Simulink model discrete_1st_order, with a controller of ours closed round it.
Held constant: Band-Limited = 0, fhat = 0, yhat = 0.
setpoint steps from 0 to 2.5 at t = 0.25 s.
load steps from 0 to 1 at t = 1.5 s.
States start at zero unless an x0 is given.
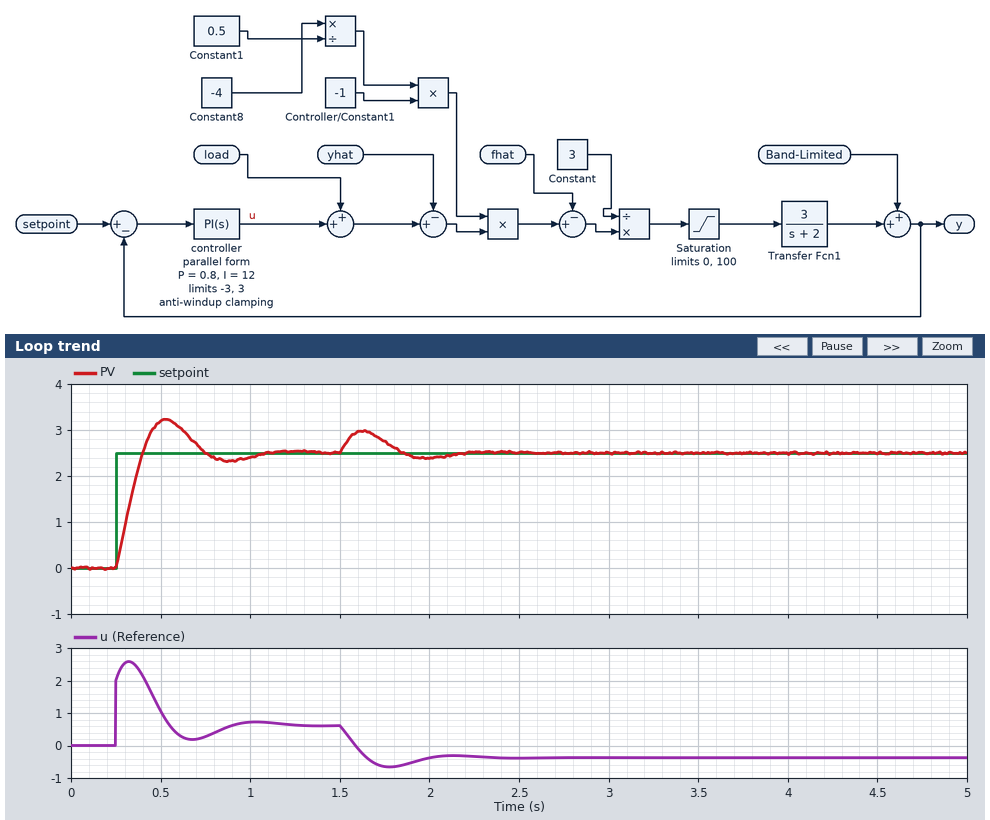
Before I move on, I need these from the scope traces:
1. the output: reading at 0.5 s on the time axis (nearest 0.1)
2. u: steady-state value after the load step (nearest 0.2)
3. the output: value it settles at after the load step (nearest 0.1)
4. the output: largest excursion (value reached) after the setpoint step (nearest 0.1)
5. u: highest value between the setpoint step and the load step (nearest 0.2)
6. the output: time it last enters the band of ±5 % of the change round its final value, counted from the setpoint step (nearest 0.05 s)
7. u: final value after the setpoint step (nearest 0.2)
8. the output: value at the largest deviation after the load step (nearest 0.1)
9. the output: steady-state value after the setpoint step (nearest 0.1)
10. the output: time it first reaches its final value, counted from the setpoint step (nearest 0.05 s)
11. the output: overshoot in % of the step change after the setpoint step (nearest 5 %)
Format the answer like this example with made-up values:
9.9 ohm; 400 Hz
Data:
3.2; -0.4; 2.5; 3.2; 2.6; 0.70 s; 0.6; 3.0; 2.5; 0.15 s; 30 %
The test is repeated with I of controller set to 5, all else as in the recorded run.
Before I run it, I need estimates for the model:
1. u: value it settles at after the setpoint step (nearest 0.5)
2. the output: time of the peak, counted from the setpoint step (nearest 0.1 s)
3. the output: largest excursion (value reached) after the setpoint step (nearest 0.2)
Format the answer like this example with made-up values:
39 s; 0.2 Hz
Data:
0.5; 0.4 s; 2.8
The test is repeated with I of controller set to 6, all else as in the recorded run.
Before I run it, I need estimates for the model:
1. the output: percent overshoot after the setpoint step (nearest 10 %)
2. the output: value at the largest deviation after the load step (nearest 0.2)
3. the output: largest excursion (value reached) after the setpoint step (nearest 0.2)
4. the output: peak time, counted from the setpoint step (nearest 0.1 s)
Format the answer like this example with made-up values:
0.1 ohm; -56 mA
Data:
20 %; 3.0; 3.0; 0.4 s
